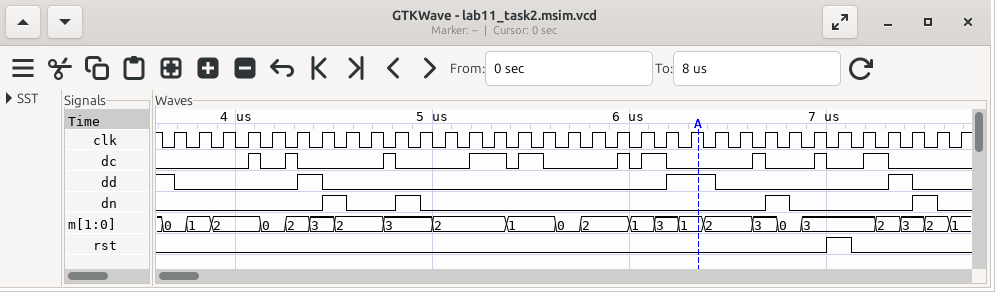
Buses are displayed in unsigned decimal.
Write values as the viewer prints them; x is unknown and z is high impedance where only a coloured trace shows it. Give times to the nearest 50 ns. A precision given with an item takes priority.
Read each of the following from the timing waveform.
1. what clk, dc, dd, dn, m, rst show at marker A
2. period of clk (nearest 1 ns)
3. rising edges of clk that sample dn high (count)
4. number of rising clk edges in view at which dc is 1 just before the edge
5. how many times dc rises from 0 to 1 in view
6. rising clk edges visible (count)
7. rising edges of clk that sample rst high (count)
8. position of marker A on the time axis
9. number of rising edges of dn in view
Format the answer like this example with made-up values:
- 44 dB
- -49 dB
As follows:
- clk=1, dc=0, dd=1, dn=0, m=1, rst=0
- 125 ns
- 4
- 7
- 10
- 33
- 1
- 6350 ns
- 4
